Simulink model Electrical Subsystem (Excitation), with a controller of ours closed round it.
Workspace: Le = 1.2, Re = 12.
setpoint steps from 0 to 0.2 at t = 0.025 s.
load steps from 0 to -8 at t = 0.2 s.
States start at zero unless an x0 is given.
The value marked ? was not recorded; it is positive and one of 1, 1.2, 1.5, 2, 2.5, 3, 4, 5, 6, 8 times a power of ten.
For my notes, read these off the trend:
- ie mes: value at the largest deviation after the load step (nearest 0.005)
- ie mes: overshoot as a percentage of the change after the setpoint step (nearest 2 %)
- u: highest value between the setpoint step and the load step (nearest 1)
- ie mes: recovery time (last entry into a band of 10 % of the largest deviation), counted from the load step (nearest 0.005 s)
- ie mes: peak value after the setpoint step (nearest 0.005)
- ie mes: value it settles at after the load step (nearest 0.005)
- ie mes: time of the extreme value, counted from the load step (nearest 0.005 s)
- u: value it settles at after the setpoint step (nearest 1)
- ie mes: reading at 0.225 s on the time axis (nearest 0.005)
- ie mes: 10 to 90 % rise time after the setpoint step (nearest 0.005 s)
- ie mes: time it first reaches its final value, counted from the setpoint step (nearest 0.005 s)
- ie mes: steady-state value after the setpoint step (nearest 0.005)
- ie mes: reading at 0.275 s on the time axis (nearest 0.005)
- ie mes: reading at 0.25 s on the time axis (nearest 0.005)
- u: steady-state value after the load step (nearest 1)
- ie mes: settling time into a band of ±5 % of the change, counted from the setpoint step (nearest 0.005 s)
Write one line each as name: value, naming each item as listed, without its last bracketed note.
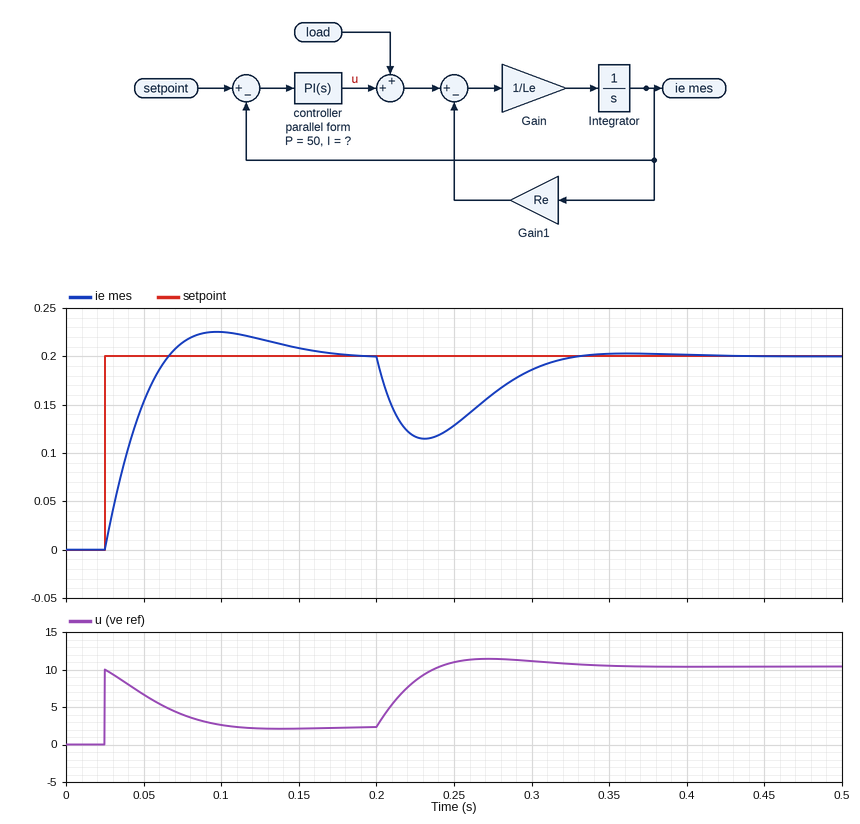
ie mes: value at the largest deviation after the load step: 0.115
ie mes: overshoot as a percentage of the change after the setpoint step: 12 %
u: highest value between the setpoint step and the load step: 10
ie mes: recovery time (last entry into a band of 10 % of the largest deviation), counted from the load step: 0.110 s
ie mes: peak value after the setpoint step: 0.225
ie mes: value it settles at after the load step: 0.200
ie mes: time of the extreme value, counted from the load step: 0.030 s
u: value it settles at after the setpoint step: 2
ie mes: reading at 0.225 s on the time axis: 0.115
ie mes: 10 to 90 % rise time after the setpoint step: 0.030 s
ie mes: time it first reaches its final value, counted from the setpoint step: 0.040 s
ie mes: steady-state value after the setpoint step: 0.200
ie mes: reading at 0.275 s on the time axis: 0.160
ie mes: reading at 0.25 s on the time axis: 0.130
u: steady-state value after the load step: 10
ie mes: settling time into a band of ±5 % of the change, counted from the setpoint step: 0.120 s
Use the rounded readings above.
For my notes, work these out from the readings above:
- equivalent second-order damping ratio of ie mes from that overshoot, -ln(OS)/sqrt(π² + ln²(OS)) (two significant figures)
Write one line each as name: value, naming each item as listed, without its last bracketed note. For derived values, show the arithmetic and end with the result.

equivalent second-order damping ratio of ie mes from that overshoot, -ln(OS)/sqrt(π² + ln²(OS)): ln(0.12) = -2.120; 2.120 / sqrt(9.870 + 4.496) = 0.56
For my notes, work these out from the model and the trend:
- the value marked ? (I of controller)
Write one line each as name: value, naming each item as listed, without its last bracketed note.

the value marked ?: 1500
